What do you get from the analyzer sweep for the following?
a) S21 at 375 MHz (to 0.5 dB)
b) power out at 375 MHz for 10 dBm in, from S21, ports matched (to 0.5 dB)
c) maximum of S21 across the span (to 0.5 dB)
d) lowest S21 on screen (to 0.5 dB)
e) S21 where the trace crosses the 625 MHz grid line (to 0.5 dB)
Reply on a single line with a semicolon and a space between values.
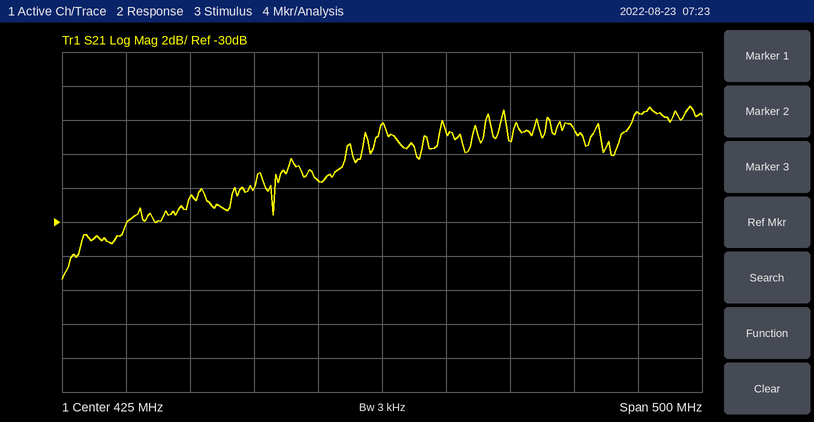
-27.5 dB; -17.5 dBm; -23.0 dB; -33.5 dB; -23.5 dB
